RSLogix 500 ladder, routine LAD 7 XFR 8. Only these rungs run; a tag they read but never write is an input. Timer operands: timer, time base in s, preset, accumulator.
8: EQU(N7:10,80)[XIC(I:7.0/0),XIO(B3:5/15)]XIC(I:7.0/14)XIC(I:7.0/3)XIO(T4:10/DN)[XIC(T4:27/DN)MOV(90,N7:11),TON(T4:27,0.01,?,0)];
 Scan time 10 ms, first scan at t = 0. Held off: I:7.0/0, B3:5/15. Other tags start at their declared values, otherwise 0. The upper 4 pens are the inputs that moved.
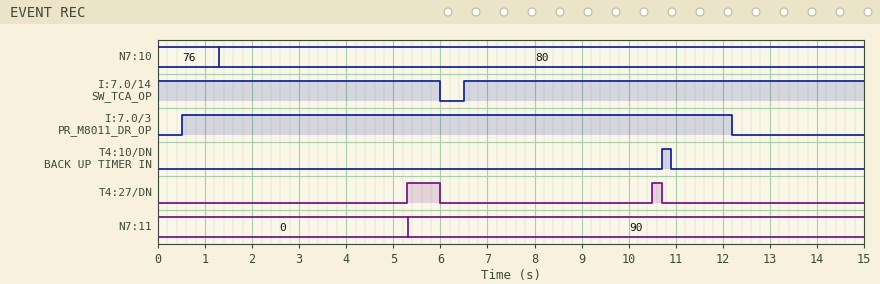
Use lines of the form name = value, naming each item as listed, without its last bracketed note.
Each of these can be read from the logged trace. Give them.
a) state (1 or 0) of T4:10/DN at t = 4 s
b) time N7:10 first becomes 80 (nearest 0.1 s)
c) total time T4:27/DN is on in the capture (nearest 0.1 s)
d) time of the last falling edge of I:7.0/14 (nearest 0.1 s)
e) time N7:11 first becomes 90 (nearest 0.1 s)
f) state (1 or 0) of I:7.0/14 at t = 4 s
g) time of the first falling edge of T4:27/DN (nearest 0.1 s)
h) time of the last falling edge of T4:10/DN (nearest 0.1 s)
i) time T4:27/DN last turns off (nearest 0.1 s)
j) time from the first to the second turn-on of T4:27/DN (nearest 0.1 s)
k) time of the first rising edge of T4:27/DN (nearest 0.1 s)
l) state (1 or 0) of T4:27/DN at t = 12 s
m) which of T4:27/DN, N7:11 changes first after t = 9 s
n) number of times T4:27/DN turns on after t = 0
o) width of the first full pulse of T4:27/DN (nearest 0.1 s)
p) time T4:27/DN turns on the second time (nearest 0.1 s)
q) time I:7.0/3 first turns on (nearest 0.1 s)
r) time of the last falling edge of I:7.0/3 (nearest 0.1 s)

state (1 or 0) of T4:10/DN at t = 4 s = 0
time N7:10 first becomes 80 = 1.3 s
total time T4:27/DN is on in the capture = 0.9 s
time of the last falling edge of I:7.0/14 = 6.0 s
time N7:11 first becomes 90 = 5.3 s
state (1 or 0) of I:7.0/14 at t = 4 s = 1
time of the first falling edge of T4:27/DN = 6.0 s
time of the last falling edge of T4:10/DN = 10.9 s
time T4:27/DN last turns off = 10.7 s
time from the first to the second turn-on of T4:27/DN = 5.2 s
time of the first rising edge of T4:27/DN = 5.3 s
state (1 or 0) of T4:27/DN at t = 12 s = 0
which of T4:27/DN, N7:11 changes first after t = 9 s = T4:27/DN
number of times T4:27/DN turns on after t = 0 = 2
width of the first full pulse of T4:27/DN = 0.7 s
time T4:27/DN turns on the second time = 10.5 s
time I:7.0/3 first turns on = 0.5 s
time of the last falling edge of I:7.0/3 = 12.2 s
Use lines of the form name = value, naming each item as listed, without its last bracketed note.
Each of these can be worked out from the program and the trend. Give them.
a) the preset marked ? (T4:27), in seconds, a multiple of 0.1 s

the preset marked ? (T4:27), in seconds, a multiple of 0.1 s = 4.0 s
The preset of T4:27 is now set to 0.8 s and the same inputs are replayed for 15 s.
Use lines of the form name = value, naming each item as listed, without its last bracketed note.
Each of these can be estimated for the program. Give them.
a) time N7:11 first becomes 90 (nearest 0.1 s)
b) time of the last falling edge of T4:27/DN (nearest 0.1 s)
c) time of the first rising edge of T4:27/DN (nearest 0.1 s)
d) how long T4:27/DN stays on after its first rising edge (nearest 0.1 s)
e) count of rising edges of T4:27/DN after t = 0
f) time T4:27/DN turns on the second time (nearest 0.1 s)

time N7:11 first becomes 90 = 2.1 s
time of the last falling edge of T4:27/DN = 12.2 s
time of the first rising edge of T4:27/DN = 2.1 s
how long T4:27/DN stays on after its first rising edge = 3.9 s
count of rising edges of T4:27/DN after t = 0 = 3
time T4:27/DN turns on the second time = 7.3 s
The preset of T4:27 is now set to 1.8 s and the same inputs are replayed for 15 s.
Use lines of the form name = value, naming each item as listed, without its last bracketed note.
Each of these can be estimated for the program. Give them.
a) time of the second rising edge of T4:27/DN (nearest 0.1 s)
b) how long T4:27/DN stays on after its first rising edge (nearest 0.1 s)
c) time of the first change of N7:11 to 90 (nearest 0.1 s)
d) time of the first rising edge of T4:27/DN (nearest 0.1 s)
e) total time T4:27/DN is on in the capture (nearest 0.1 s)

time of the second rising edge of T4:27/DN = 8.3 s
how long T4:27/DN stays on after its first rising edge = 2.9 s
time of the first change of N7:11 to 90 = 3.1 s
time of the first rising edge of T4:27/DN = 3.1 s
total time T4:27/DN is on in the capture = 5.3 s
